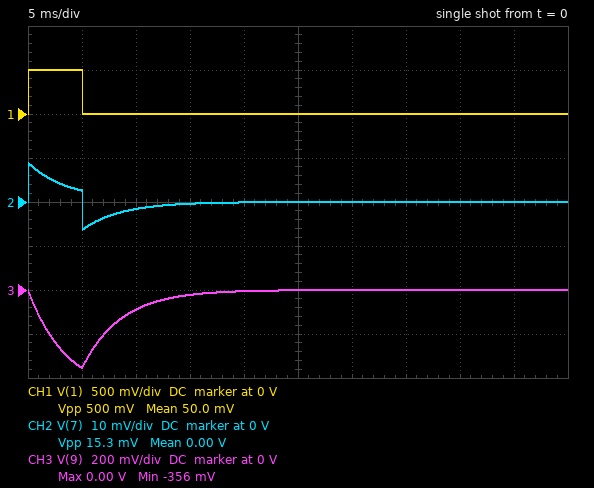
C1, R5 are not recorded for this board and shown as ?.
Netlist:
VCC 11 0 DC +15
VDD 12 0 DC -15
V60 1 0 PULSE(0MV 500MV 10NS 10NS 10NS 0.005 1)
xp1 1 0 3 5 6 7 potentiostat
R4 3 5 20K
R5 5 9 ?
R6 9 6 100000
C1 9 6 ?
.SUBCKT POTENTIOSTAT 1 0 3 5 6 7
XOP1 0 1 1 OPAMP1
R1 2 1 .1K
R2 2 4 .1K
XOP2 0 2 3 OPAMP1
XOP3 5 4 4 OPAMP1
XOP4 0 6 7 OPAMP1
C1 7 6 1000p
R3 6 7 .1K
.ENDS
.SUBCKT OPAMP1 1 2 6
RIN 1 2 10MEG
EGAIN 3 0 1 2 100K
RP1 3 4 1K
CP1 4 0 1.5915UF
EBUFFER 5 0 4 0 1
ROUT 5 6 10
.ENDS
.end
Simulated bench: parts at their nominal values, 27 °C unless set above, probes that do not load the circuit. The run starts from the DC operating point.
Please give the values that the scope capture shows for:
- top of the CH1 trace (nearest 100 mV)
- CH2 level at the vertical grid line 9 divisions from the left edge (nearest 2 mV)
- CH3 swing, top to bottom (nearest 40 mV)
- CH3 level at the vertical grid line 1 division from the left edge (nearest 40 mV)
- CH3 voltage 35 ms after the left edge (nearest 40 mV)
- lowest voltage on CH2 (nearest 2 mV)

500 mV
0 V
360 mV
-360 mV
0 V
-6 mV
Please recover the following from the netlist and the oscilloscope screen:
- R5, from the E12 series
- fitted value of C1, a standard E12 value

5.6 kΩ
680 nF
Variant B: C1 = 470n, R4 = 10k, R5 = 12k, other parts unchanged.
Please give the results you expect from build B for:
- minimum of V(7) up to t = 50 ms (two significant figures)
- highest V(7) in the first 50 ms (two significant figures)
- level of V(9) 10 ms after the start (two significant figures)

-2.3 mV
4.2 mV
-100 mV
